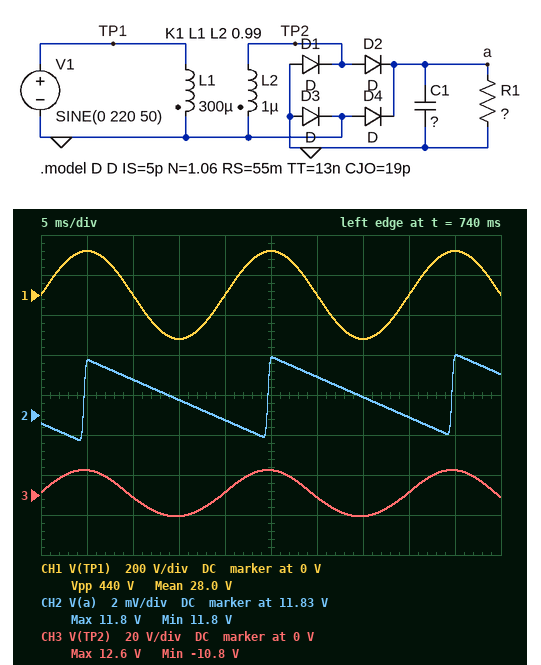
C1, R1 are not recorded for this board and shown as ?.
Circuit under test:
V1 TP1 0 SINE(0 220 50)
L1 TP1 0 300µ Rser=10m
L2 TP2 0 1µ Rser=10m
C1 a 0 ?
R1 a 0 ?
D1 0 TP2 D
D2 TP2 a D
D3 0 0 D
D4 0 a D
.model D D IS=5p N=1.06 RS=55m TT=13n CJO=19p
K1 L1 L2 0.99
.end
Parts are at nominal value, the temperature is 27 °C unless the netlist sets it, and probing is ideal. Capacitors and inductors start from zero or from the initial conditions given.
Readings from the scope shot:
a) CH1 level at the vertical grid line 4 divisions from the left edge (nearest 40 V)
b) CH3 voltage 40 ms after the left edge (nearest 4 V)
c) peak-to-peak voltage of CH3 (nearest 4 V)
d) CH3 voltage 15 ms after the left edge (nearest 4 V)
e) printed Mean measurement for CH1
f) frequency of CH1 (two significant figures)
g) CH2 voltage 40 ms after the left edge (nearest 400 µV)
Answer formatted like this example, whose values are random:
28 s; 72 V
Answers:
0 V; 0 V; 24 V; -12 V; 28.0 V; 50 Hz; 11.8300 V
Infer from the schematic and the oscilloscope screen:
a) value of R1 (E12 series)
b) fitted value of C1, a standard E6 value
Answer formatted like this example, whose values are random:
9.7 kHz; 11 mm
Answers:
3.9 kΩ; 15 mF
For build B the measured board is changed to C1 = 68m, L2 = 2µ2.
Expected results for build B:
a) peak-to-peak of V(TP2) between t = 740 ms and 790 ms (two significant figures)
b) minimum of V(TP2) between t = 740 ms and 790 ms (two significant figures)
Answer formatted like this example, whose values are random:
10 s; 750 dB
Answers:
34 V; -16 V
